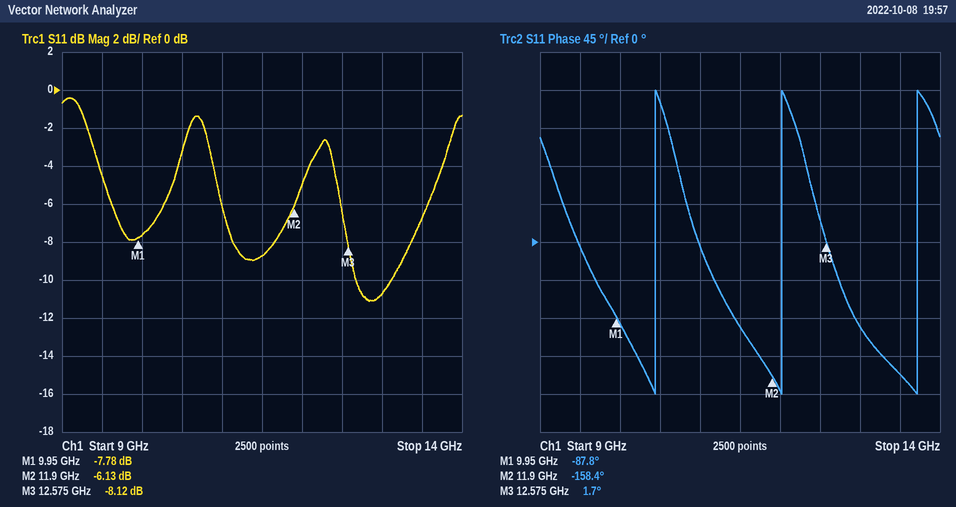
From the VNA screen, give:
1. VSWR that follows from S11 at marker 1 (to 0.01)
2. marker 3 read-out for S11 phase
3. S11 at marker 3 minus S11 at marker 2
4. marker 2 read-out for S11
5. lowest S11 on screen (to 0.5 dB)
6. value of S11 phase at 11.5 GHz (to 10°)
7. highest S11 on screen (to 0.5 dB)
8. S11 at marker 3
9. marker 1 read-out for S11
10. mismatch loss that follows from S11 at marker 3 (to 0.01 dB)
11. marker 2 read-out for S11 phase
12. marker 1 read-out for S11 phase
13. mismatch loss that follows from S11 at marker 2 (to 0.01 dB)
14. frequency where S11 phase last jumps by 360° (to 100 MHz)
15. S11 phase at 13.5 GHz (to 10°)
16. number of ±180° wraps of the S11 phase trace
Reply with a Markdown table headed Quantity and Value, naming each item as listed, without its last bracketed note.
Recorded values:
| Quantity | Value |
|---|---|
| VSWR that follows from S11 at marker 1 | 2.38 |
| marker 3 read-out for S11 phase | 1.7° |
| S11 at marker 3 minus S11 at marker 2 | -1.99 dB |
| marker 2 read-out for S11 | -6.13 dB |
| lowest S11 on screen | -11.0 dB |
| value of S11 phase at 11.5 GHz | -100° |
| highest S11 on screen | -0.5 dB |
| S11 at marker 3 | -8.12 dB |
| marker 1 read-out for S11 | -7.78 dB |
| mismatch loss that follows from S11 at marker 3 | 0.73 dB |
| marker 2 read-out for S11 phase | -158.4° |
| marker 1 read-out for S11 phase | -87.8° |
| mismatch loss that follows from S11 at marker 2 | 1.21 dB |
| frequency where S11 phase last jumps by 360° | 13.7 GHz |
| S11 phase at 13.5 GHz | -160° |
| number of ±180° wraps of the S11 phase trace | 3 |
